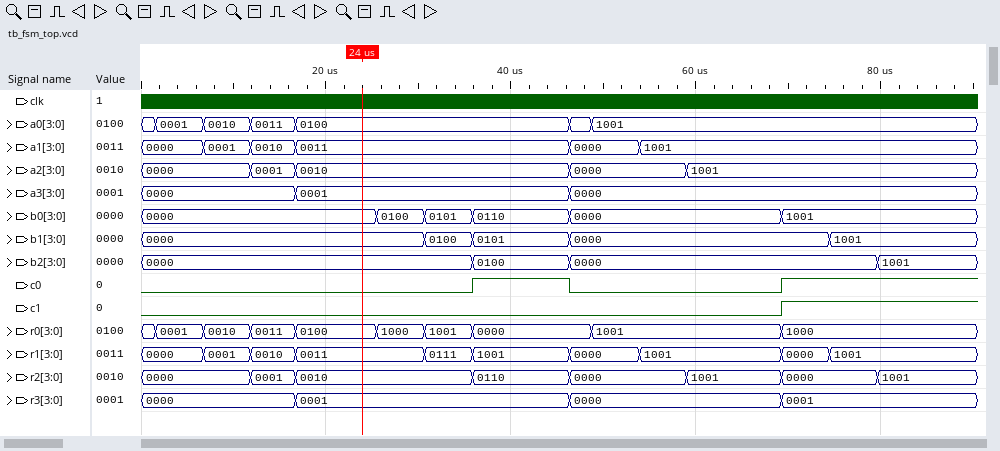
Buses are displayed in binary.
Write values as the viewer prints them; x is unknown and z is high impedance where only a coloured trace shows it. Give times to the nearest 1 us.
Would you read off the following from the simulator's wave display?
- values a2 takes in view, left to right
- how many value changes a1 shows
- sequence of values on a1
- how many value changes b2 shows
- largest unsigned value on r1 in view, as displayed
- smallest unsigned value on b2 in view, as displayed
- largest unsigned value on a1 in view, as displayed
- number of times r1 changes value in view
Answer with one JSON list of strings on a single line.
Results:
["0000, 0001, 0010, 0000, 1001", "5", "0000, 0001, 0010, 0011, 0000, 1001", "3", "1001", "0000", "1001", "9"]
